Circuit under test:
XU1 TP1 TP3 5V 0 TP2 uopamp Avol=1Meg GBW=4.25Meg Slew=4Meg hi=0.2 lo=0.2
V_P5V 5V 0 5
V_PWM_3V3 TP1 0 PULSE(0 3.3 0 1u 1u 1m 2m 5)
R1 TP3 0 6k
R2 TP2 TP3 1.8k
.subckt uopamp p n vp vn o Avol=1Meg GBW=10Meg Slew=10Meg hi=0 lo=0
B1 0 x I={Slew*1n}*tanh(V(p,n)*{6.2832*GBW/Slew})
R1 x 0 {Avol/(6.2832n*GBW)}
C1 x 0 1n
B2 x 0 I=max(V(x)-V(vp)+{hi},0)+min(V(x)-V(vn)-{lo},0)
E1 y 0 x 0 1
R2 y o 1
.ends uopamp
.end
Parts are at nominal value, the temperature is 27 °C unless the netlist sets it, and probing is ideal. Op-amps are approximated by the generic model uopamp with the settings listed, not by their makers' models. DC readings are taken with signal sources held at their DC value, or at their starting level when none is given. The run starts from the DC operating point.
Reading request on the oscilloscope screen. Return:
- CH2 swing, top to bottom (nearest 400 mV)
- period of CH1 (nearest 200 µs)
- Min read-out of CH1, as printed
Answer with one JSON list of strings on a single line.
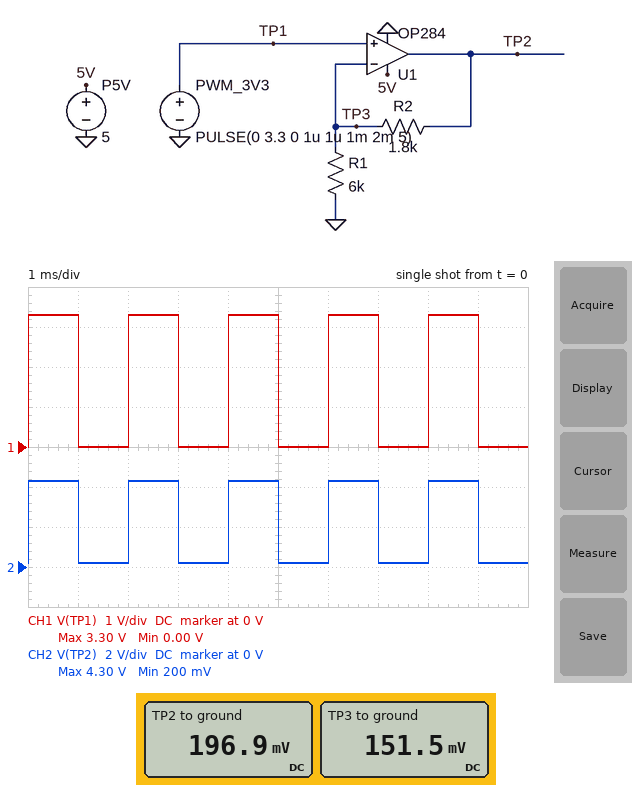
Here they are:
["4.0 V", "2.0 ms", "0.00 V"]
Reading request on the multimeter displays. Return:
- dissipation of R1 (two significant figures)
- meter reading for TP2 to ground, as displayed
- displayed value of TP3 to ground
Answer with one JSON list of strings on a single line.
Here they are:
["3.8 µW", "196.9 mV", "151.5 mV"]
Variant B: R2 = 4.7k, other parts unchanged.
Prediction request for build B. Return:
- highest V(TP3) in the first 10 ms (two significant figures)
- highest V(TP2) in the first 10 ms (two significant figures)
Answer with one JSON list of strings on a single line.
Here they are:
["2.7 V", "4.8 V"]
